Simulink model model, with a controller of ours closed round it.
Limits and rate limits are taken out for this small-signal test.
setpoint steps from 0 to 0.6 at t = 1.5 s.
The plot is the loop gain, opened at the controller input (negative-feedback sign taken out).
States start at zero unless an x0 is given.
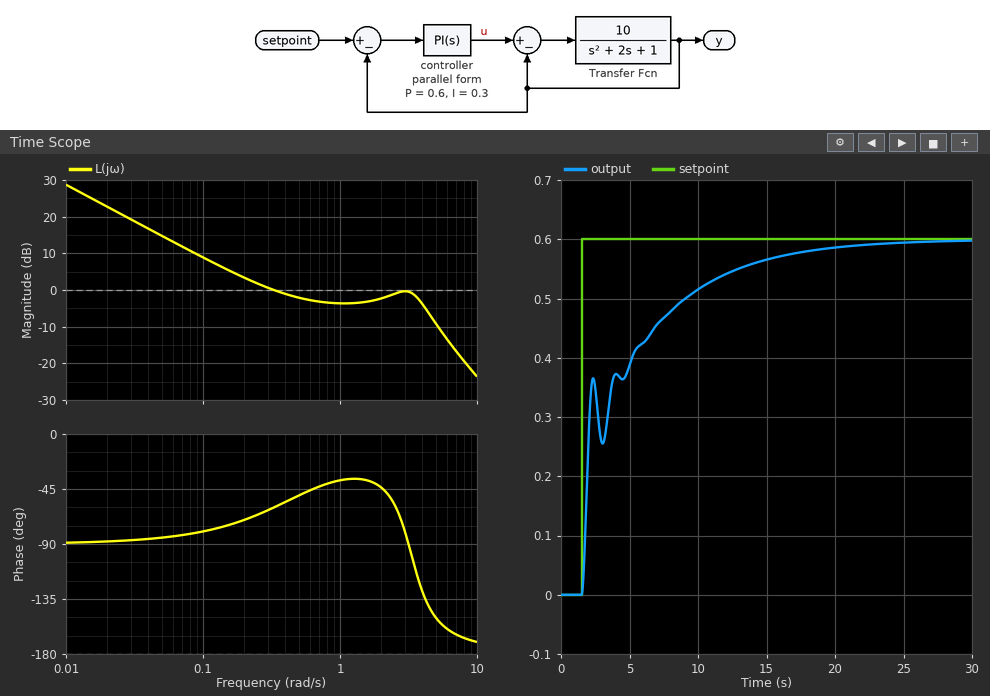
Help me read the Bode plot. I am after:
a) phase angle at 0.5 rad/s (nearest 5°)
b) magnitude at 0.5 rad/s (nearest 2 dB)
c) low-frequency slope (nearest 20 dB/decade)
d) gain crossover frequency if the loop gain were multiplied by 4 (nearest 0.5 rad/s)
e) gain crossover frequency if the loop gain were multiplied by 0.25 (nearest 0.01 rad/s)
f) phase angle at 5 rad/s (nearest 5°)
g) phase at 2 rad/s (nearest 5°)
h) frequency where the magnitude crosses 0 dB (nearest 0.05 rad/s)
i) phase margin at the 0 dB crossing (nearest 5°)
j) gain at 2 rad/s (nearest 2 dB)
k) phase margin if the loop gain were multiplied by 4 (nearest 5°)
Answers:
-50°
-2 dB
-20 dB/decade
5.5 rad/s
0.07 rad/s
-150°
-45°
0.35 rad/s
120°
-2 dB
25°
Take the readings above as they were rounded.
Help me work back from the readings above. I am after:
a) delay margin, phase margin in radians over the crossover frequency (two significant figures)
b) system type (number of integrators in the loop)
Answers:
6.0 s
1
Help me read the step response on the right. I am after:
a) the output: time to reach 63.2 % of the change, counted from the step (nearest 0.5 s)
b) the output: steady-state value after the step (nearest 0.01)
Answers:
3.5 s
0.60
